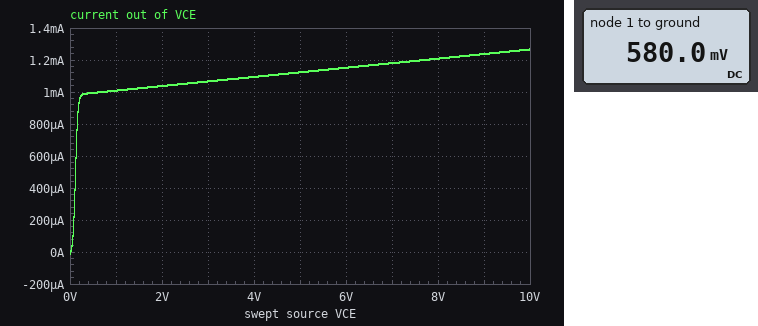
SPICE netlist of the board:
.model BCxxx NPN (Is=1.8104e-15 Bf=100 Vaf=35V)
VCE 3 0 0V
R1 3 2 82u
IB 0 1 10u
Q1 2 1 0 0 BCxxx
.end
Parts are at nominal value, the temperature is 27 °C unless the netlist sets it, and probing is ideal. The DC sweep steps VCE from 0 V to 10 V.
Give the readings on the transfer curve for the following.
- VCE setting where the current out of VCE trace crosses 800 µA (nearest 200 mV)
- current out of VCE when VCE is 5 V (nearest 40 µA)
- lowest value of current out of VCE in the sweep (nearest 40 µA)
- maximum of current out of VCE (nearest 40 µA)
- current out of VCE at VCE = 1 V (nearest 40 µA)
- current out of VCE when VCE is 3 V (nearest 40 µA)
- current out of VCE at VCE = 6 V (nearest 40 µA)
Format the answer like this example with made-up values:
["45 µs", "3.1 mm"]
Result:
["200 mV", "1.12 mA", "0 A", "1.28 mA", "1.00 mA", "1.08 mA", "1.16 mA"]
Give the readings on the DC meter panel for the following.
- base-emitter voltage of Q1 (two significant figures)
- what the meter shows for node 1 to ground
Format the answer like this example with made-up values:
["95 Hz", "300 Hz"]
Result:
["580 mV", "580.0 mV"]
